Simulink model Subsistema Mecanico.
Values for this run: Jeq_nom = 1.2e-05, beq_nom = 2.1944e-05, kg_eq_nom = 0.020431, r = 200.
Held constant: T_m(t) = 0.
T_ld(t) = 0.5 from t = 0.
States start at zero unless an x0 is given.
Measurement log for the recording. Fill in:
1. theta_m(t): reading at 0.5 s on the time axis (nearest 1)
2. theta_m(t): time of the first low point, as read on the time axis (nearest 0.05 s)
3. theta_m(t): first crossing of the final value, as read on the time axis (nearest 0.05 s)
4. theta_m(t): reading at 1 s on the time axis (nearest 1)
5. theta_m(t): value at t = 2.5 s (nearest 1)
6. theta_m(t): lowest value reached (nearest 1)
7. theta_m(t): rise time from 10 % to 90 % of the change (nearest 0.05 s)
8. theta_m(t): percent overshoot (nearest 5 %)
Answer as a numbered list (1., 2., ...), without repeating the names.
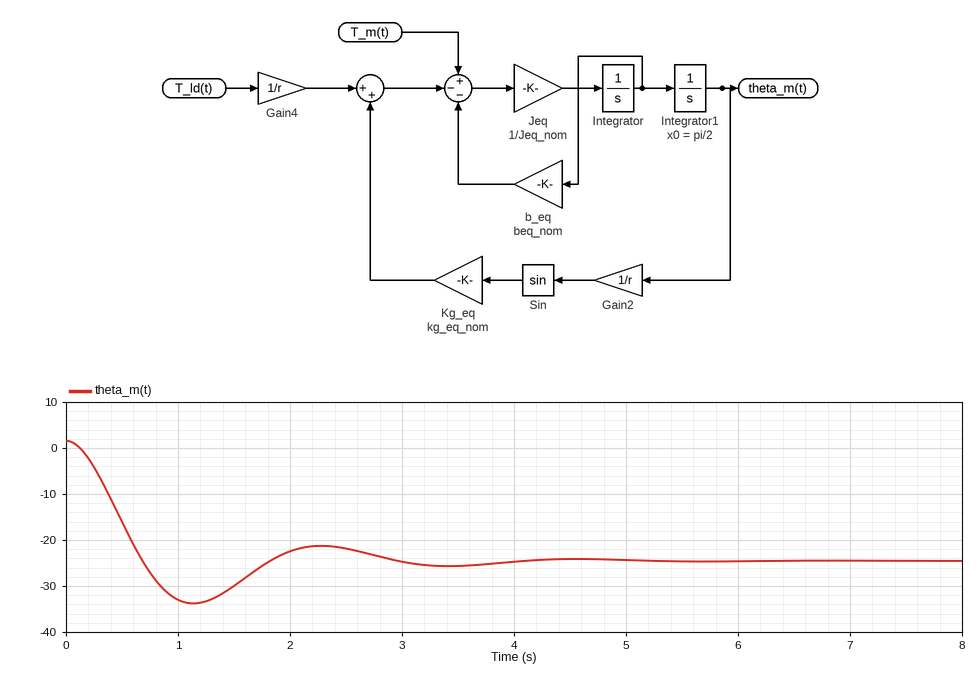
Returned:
1. -16
2. 1.15 s
3. 0.70 s
4. -33
5. -22
6. -34
7. 0.45 s
8. 35 %
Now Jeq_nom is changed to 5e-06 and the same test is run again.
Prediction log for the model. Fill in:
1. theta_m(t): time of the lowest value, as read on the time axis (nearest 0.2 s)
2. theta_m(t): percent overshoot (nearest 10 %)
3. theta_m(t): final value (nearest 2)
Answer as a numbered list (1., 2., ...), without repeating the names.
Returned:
1. 0.8 s
2. 20 %
3. -24
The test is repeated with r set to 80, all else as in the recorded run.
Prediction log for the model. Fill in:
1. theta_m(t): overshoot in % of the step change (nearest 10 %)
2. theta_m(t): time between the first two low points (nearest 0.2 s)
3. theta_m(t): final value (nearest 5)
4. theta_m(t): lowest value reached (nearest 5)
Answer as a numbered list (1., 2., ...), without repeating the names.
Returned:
1. 50 %
2. 1.4 s
3. -25
4. -40
